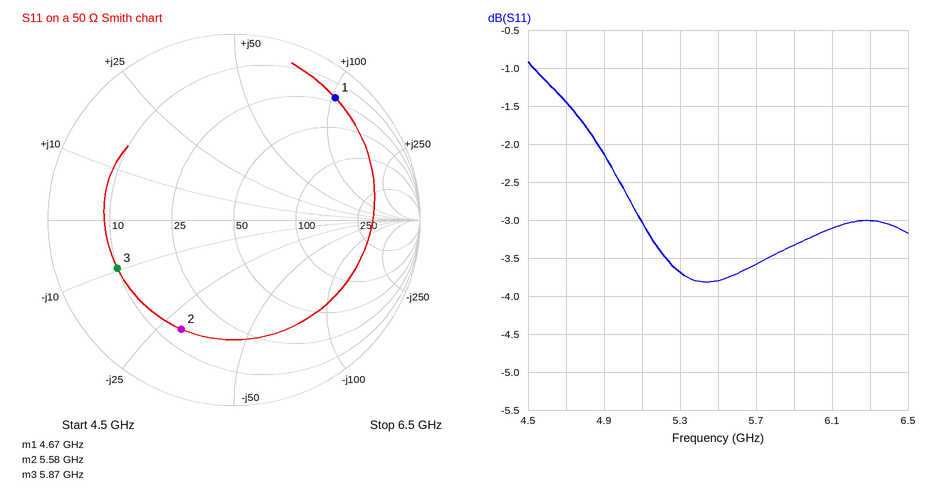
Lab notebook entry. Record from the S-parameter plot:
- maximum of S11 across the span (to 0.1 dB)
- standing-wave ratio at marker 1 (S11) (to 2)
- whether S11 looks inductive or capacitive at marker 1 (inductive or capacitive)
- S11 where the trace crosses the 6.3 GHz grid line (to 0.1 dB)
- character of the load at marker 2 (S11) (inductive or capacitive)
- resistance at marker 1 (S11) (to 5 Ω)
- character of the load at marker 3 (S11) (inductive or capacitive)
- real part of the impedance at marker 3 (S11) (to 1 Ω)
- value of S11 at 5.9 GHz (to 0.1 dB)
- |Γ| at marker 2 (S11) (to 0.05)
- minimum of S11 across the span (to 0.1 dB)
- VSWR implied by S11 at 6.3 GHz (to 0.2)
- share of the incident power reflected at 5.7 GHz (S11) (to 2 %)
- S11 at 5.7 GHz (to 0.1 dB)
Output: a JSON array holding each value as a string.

["-0.9 dB", "12", "inductive", "-3.0 dB", "capacitive", "20 Ω", "capacitive", "10 Ω", "-3.3 dB", "0.65", "-3.8 dB", "5.8", "44 %", "-3.6 dB"]
